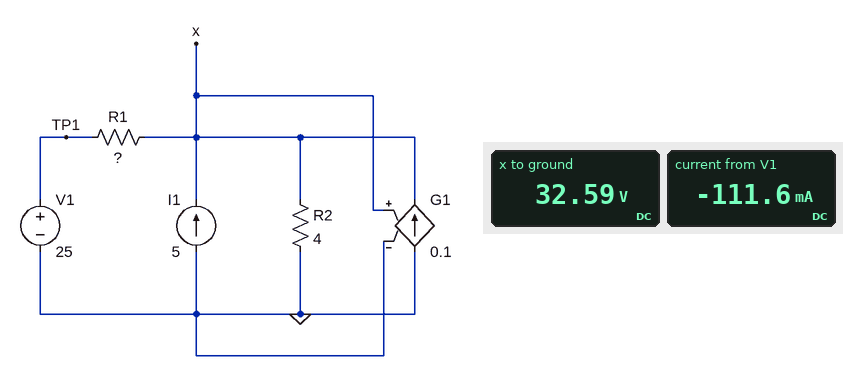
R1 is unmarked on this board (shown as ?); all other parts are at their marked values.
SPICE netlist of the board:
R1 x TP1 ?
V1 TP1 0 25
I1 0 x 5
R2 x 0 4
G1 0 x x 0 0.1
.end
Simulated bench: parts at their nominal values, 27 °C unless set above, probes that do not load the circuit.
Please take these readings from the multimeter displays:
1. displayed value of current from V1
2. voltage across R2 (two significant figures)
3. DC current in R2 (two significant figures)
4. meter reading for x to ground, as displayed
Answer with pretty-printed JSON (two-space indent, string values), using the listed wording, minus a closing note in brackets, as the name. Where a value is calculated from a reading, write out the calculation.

{
  "displayed value of current from V1": "-111.6 mA",
  "voltage across R2": "32.59 V = 33 V",
  "DC current in R2": "(32.59 V) / 4 Ω = 8.1 A",
  "meter reading for x to ground, as displayed": "32.59 V"
}
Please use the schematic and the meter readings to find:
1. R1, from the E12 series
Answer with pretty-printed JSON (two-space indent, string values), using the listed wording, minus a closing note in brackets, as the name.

{
  "R1, from the E12 series": "68 Ω"
}
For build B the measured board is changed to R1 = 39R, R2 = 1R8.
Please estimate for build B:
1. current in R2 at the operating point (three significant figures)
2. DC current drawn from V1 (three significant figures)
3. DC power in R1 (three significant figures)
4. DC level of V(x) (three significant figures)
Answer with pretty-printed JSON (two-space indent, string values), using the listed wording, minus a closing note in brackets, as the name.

{
  "current in R2 at the operating point": "6.51 A",
  "DC current drawn from V1": "340 mA",
  "DC power in R1": "4.52 W",
  "DC level of V(x)": "11.7 V"
}
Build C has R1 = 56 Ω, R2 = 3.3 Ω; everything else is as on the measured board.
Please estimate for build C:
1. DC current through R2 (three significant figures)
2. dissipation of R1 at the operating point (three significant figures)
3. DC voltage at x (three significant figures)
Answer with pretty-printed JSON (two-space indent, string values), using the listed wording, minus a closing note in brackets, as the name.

{
  "DC current through R2": "7.47 A",
  "dissipation of R1 at the operating point": "2.10 mW",
  "DC voltage at x": "24.7 V"
}
